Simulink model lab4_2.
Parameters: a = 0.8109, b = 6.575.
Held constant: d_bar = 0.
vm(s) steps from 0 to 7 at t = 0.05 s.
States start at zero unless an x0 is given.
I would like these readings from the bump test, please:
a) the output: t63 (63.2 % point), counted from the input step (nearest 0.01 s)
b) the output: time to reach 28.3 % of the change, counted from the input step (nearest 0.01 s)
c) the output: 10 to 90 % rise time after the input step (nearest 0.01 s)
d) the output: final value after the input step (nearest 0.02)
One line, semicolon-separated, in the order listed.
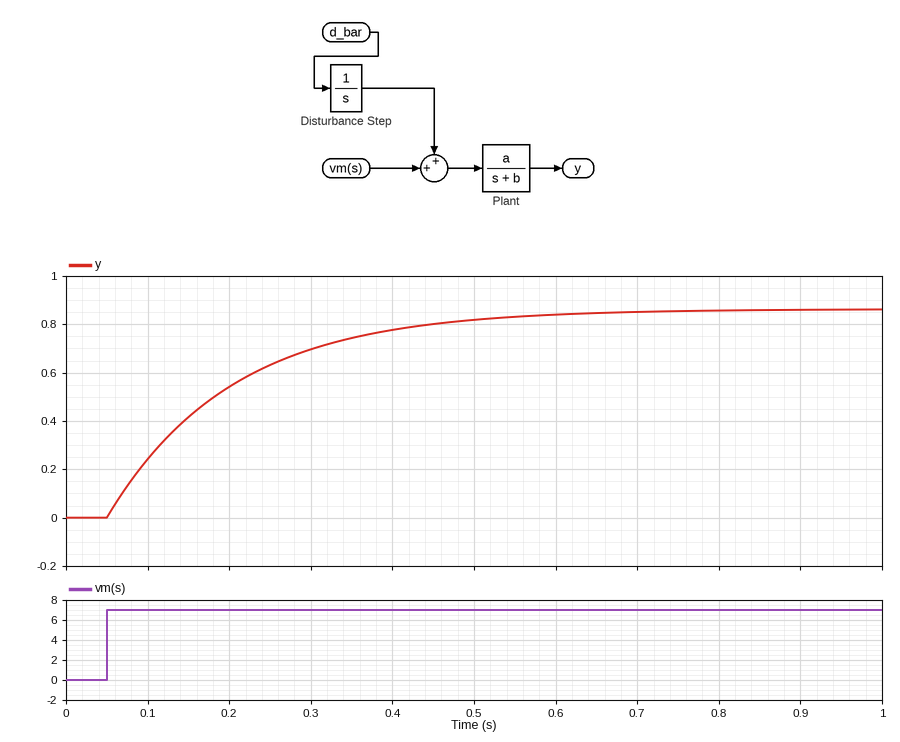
0.15 s; 0.05 s; 0.33 s; 0.86
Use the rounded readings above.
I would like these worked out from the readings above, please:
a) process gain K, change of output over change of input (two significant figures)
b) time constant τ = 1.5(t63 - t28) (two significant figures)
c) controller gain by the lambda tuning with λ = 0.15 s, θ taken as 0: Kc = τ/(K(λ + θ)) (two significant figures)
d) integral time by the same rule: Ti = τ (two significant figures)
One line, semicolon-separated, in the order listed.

0.12; 0.15 s; 8.3; 0.15 s
